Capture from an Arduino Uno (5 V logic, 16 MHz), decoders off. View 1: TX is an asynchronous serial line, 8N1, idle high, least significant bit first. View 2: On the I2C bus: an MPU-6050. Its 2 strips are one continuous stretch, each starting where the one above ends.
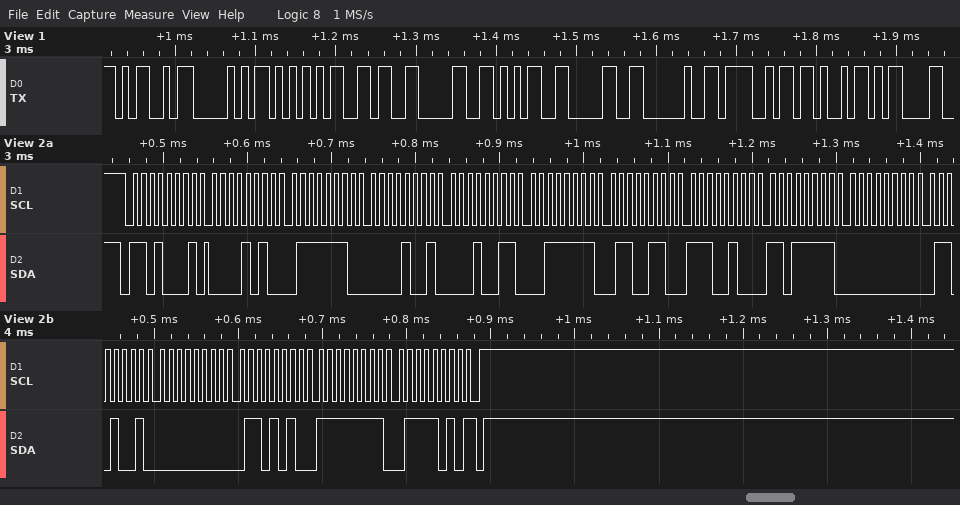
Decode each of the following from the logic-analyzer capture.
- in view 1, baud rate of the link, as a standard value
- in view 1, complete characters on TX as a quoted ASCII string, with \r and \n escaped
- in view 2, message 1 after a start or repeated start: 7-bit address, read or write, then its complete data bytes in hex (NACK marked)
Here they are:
115200 baud
"MPU6050 OK\r"
0x68 read: 0A 7E 09 13 3F 66 E4 DF 00 69 00 6A FF 7A NACK
